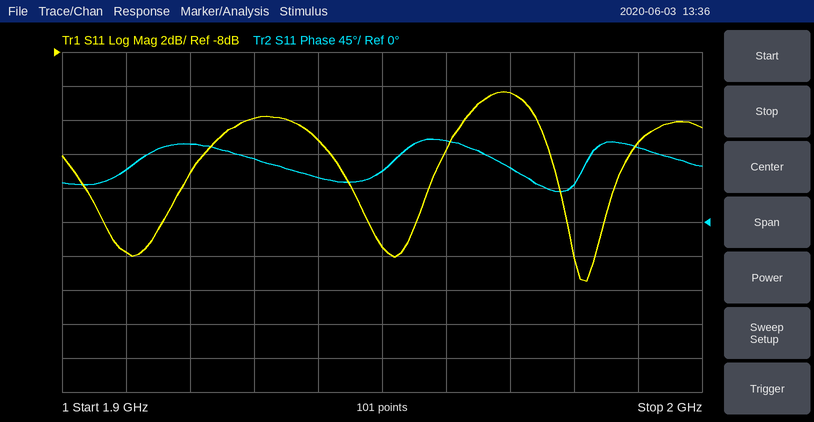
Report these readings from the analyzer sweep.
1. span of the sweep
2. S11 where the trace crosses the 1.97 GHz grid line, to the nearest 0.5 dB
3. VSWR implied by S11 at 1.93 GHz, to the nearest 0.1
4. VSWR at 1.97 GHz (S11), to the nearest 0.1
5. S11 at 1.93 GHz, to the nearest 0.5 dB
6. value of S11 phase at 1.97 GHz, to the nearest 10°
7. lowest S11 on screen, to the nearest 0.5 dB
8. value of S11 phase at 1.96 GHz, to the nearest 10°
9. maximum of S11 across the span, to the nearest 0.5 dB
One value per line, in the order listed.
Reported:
100 MHz
-10.5 dB
1.7
1.9
-12.0 dB
70°
-21.5 dB
110°
-10.5 dB
